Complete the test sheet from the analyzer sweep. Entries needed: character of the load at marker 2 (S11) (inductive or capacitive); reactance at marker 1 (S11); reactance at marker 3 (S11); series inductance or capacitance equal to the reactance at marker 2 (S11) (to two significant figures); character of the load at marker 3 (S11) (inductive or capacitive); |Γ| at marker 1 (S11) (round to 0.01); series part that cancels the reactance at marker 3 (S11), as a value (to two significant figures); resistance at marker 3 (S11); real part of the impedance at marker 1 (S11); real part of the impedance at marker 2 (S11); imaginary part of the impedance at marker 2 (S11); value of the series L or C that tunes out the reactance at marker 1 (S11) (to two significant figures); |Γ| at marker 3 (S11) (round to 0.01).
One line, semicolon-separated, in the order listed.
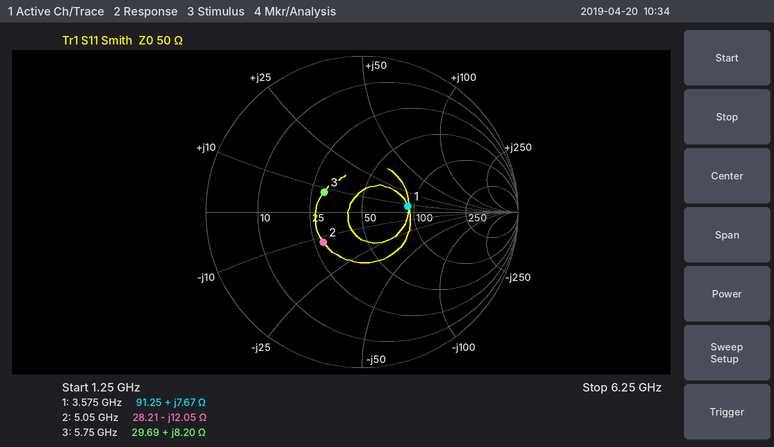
capacitive; +7.67 Ω; +8.20 Ω; 2.6 pF; inductive; 0.30; 3.4 pF; 29.69 Ω; 91.25 Ω; 28.21 Ω; -12.05 Ω; 5.8 pF; 0.27
